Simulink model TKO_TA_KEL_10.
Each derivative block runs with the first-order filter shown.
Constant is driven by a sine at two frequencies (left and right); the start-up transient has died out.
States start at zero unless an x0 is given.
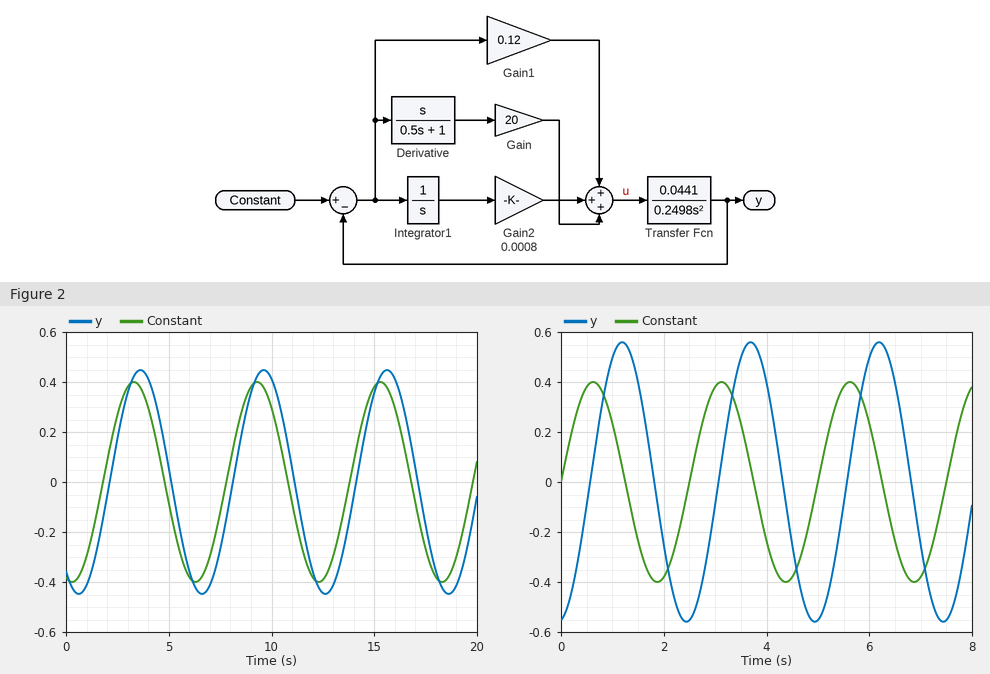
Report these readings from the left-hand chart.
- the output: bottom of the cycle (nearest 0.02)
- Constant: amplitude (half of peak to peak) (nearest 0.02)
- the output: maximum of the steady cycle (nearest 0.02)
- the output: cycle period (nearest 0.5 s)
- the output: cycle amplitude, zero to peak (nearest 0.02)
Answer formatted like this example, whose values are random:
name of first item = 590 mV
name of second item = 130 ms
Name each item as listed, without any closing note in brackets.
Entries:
the output: bottom of the cycle = -0.44
Constant: amplitude (half of peak to peak) = 0.40
the output: maximum of the steady cycle = 0.44
the output: cycle period = 6.0 s
the output: cycle amplitude, zero to peak = 0.44
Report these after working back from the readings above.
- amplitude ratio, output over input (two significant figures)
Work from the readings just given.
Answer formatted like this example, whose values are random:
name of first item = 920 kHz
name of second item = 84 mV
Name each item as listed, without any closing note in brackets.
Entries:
amplitude ratio, output over input = 1.1
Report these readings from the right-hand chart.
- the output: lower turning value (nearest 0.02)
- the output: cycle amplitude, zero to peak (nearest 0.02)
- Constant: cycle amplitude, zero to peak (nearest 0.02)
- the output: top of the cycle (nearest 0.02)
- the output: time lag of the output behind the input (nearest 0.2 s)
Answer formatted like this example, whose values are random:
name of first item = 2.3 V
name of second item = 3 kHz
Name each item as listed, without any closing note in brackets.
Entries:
the output: lower turning value = -0.56
the output: cycle amplitude, zero to peak = 0.56
Constant: cycle amplitude, zero to peak = 0.40
the output: top of the cycle = 0.56
the output: time lag of the output behind the input = 0.6 s
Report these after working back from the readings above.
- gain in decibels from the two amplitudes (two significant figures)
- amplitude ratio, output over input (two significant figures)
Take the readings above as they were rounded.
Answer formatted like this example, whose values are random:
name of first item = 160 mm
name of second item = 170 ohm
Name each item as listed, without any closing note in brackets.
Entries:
gain in decibels from the two amplitudes = 2.9 dB
amplitude ratio, output over input = 1.4
